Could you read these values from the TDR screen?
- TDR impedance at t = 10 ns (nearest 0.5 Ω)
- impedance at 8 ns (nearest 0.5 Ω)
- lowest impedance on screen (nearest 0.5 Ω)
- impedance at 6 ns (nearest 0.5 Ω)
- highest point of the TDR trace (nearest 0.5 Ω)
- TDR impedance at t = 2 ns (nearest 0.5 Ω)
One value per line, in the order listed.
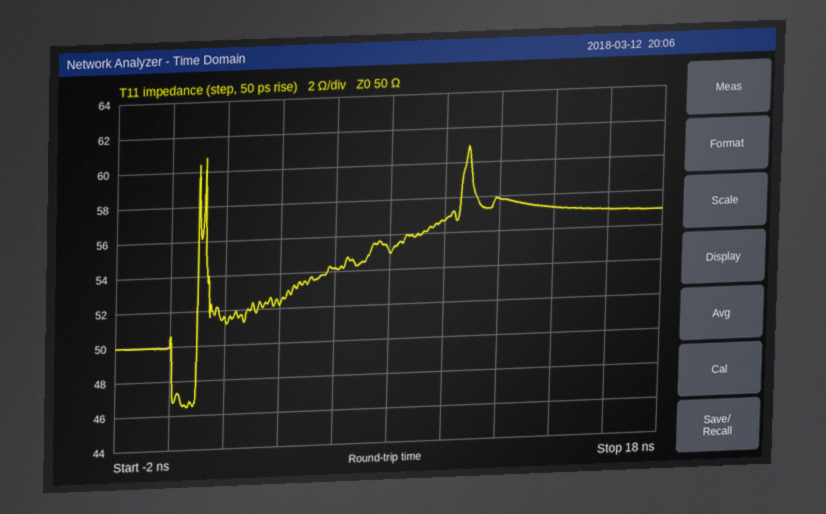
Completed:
56.5 Ω
55.0 Ω
46.5 Ω
54.0 Ω
61.0 Ω
51.5 Ω
